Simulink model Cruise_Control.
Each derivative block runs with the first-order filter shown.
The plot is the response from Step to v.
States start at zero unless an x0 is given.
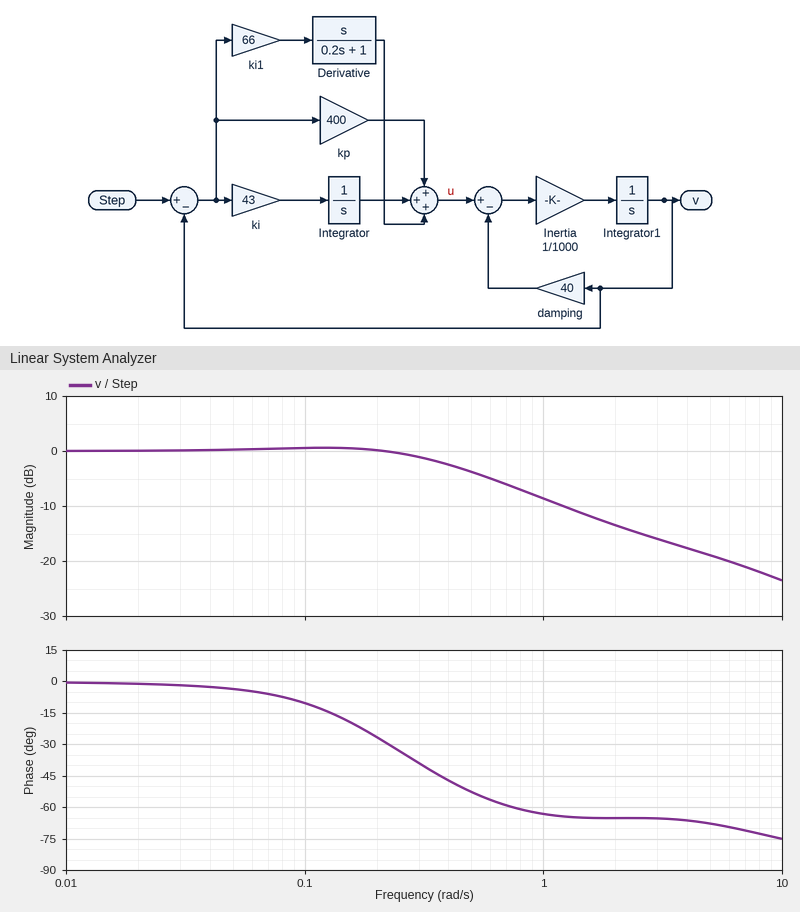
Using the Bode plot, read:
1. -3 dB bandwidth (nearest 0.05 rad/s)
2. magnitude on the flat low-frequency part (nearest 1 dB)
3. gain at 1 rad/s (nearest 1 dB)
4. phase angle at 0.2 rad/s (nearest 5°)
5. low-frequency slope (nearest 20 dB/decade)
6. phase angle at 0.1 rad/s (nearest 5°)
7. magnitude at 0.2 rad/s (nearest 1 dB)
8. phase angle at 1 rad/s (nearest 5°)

0.45 rad/s
0 dB
-9 dB
-25°
0 dB/decade
-10°
0 dB
-65°
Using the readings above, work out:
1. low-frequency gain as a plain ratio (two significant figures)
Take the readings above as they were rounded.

1.0
